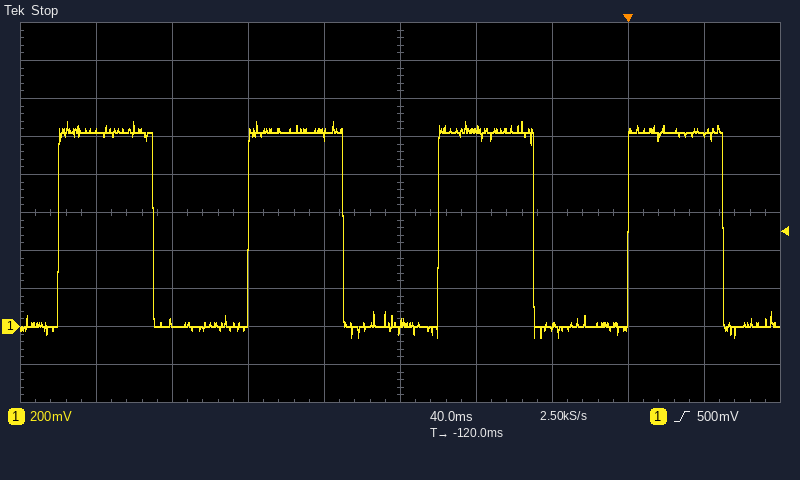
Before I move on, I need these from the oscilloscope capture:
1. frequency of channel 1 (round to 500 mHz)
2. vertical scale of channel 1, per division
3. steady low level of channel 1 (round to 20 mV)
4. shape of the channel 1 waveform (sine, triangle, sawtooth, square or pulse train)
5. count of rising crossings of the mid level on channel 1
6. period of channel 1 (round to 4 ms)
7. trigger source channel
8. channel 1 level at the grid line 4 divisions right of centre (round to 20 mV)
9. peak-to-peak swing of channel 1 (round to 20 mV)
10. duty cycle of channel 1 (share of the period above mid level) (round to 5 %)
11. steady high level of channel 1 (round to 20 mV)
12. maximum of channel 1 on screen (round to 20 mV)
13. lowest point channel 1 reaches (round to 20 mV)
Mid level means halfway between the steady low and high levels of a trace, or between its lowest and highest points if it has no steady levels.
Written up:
10.0 Hz
200 mV
0 mV
square
4
100 ms
channel 1
1.02 V
1.14 V
50 %
1.02 V
1.08 V
-60 mV
